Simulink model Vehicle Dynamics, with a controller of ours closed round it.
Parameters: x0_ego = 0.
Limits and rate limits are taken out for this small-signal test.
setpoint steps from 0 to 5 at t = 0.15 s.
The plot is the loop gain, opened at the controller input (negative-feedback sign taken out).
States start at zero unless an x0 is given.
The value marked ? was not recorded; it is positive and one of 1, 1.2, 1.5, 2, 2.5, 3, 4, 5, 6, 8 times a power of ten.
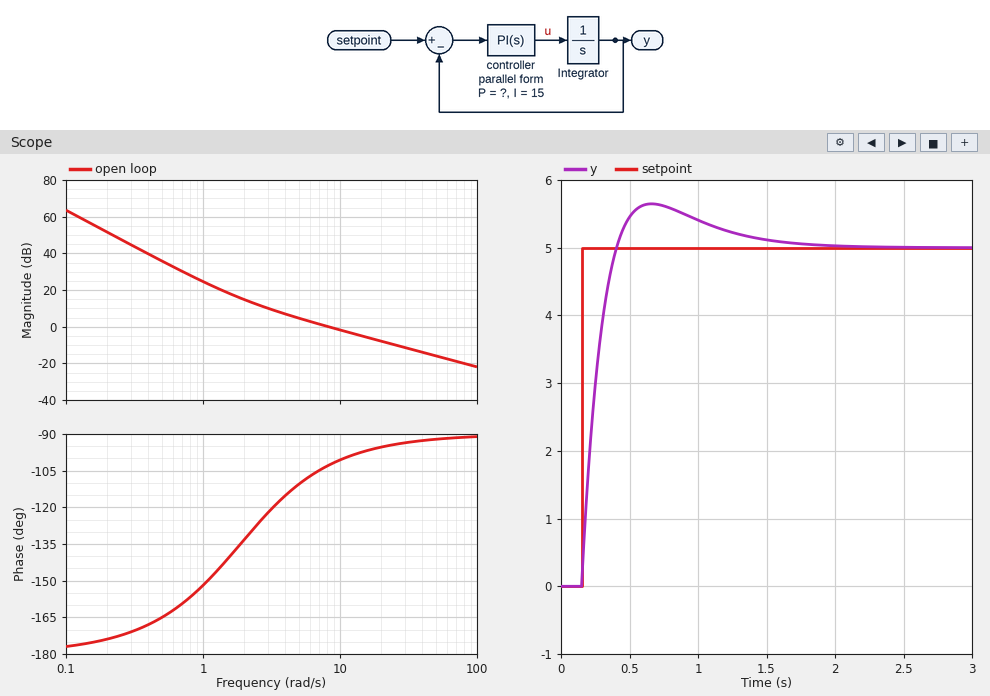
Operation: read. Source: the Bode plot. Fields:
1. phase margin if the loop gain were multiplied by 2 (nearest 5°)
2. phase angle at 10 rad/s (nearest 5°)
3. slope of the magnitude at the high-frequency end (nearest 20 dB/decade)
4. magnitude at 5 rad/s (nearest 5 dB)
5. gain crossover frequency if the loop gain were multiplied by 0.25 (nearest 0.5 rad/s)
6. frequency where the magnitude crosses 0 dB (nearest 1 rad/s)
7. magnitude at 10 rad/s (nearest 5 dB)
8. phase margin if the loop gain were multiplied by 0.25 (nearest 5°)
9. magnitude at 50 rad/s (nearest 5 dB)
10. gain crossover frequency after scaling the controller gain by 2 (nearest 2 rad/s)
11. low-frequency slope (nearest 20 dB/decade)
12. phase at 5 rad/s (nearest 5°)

85°
-100°
-20 dB/decade
5 dB
2.5 rad/s
8 rad/s
0 dB
55°
-15 dB
16 rad/s
-40 dB/decade
-110°
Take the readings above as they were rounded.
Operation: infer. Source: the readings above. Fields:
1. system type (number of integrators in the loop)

2
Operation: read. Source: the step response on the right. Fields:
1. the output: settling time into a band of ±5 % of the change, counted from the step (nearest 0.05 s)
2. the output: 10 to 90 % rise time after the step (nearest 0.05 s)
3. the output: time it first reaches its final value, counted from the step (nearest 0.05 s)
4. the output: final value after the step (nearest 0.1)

1.05 s
0.20 s
0.25 s
5.0
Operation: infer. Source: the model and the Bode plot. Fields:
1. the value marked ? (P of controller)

8
